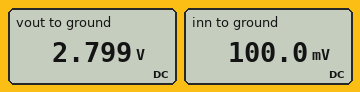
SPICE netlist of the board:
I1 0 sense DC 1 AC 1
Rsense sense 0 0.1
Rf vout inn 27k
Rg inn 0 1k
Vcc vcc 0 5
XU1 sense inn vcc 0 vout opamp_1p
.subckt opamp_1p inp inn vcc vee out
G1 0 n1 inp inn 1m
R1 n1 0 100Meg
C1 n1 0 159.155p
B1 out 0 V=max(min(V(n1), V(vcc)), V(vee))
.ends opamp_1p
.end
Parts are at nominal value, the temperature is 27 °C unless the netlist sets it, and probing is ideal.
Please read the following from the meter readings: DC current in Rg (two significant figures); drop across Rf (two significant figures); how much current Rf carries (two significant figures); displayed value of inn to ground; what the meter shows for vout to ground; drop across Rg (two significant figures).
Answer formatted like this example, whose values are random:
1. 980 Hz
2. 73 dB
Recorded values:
1. 100 µA
2. 2.7 V
3. 100 µA
4. 100.0 mV
5. 2.799 V
6. 100 mV
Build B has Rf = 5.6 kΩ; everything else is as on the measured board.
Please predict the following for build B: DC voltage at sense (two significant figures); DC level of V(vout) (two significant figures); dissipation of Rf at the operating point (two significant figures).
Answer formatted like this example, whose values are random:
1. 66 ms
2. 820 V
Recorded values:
1. 100 mV
2. 660 mV
3. 56 µW
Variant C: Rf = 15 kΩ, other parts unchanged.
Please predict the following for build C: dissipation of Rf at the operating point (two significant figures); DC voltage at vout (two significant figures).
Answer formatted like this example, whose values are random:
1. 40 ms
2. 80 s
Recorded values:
1. 150 µW
2. 1.6 V
